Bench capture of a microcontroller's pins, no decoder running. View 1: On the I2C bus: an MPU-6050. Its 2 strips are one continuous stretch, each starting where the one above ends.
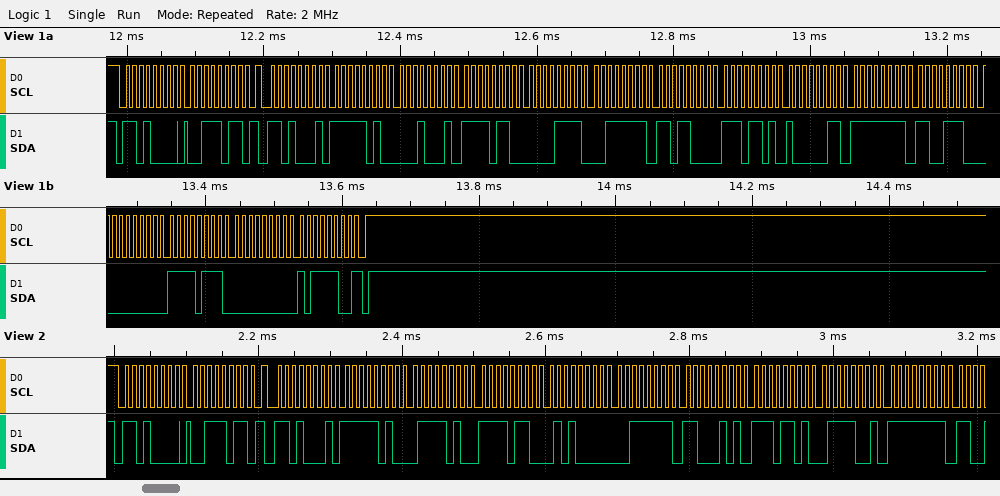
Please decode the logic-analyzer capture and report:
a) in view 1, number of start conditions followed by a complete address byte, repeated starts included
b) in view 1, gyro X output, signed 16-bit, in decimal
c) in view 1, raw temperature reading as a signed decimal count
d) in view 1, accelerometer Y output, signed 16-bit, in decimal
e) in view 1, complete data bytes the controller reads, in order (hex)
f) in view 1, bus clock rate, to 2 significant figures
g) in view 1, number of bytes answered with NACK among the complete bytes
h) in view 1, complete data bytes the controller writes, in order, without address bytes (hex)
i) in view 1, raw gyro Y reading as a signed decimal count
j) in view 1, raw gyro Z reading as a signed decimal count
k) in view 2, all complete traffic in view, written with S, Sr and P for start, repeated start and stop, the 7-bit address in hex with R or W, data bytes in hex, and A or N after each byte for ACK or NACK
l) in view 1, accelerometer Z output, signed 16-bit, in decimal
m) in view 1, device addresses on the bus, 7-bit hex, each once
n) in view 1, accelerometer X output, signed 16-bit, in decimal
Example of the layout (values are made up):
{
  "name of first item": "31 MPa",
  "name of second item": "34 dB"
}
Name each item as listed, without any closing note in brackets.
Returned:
{
  "in view 1, number of start conditions followed by a complete address byte, repeated starts included": "2",
  "in view 1, gyro X output, signed 16-bit, in decimal": "-50",
  "in view 1, raw temperature reading as a signed decimal count": "-4733",
  "in view 1, accelerometer Y output, signed 16-bit, in decimal": "-2545",
  "in view 1, complete data bytes the controller reads, in order": "FA 11 F6 0F 3F D8 ED 83 FF CE 00 F7 00 BC",
  "in view 1, bus clock rate, to 2 significant figures": "100 kHz",
  "in view 1, number of bytes answered with NACK among the complete bytes": "1",
  "in view 1, complete data bytes the controller writes, in order, without address bytes": "3B",
  "in view 1, raw gyro Y reading as a signed decimal count": "247",
  "in view 1, raw gyro Z reading as a signed decimal count": "188",
  "in view 2, all complete traffic in view, written with S, Sr and P for start, repeated start and stop, the 7-bit address in hex with R or W, data bytes in hex, and A or N after each byte for ACK or NACK": "S 68W A 3B A Sr 68R A FA A 7A A F6 A 50 A 3F A C5 A ED A 79 A FF A",
  "in view 1, accelerometer Z output, signed 16-bit, in decimal": "16344",
  "in view 1, device addresses on the bus, 7-bit hex, each once": "0x68",
  "in view 1, accelerometer X output, signed 16-bit, in decimal": "-1519"
}
